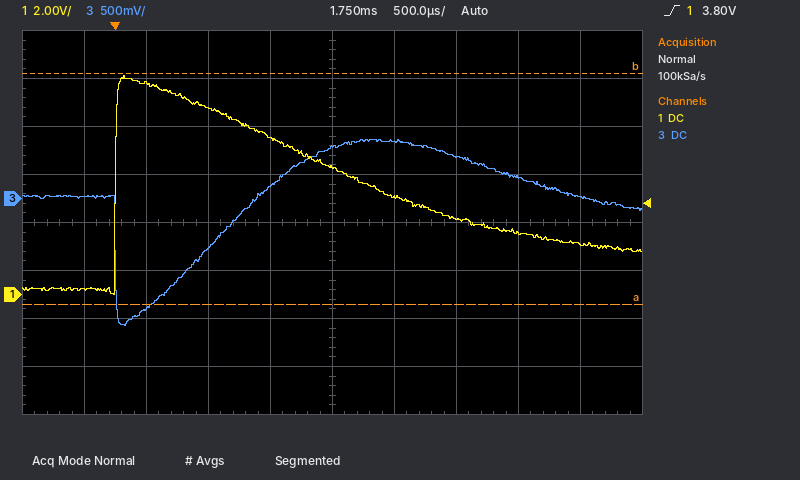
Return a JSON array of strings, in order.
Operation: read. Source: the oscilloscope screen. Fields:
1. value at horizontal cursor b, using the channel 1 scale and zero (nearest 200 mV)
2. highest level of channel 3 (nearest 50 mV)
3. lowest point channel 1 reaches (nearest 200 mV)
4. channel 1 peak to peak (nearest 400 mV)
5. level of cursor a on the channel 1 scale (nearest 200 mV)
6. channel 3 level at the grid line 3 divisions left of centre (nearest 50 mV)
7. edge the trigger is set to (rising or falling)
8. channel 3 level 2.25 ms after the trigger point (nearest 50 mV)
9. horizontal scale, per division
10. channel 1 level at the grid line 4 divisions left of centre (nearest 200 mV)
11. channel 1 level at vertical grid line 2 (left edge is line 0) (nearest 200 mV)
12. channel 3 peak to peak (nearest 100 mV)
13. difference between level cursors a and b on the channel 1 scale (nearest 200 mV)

["9.2 V", "600 mV", "0.0 V", "9.2 V", "-400 mV", "-1.15 V", "rising", "600 mV", "500 µs", "200 mV", "8.8 V", "1.90 V", "9.6 V"]
